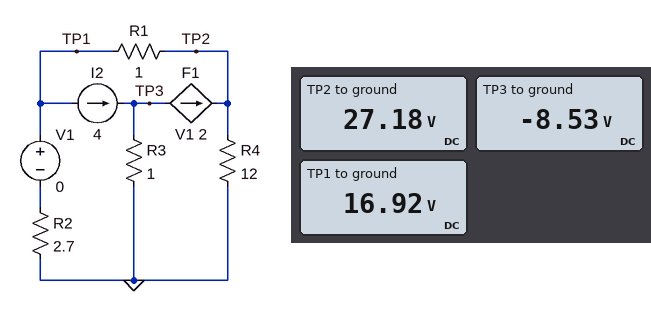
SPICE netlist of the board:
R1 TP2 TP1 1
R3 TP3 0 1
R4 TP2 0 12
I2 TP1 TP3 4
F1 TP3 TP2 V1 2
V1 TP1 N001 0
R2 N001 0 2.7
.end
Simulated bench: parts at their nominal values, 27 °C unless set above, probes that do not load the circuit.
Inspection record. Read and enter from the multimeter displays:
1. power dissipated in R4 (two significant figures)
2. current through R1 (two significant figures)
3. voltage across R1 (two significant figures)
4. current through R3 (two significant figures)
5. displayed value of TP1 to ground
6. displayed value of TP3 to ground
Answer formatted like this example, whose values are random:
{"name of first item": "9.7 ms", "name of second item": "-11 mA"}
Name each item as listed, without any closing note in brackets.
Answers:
{"power dissipated in R4": "62 W", "current through R1": "10 A", "voltage across R1": "10 V", "current through R3": "8.5 A", "displayed value of TP1 to ground": "16.92 V", "displayed value of TP3 to ground": "-8.53 V"}
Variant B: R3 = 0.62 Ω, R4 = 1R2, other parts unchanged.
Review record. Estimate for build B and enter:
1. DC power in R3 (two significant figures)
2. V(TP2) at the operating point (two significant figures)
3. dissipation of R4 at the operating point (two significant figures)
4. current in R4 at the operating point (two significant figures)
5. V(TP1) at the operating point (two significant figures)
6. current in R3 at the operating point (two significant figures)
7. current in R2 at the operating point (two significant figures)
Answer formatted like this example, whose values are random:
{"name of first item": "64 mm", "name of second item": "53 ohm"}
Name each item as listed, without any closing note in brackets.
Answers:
{"DC power in R3": "76 W", "V(TP2) at the operating point": "-9.0 V", "dissipation of R4 at the operating point": "68 W", "current in R4 at the operating point": "7.5 A", "V(TP1) at the operating point": "-9.5 V", "current in R3 at the operating point": "11 A", "current in R2 at the operating point": "3.5 A"}
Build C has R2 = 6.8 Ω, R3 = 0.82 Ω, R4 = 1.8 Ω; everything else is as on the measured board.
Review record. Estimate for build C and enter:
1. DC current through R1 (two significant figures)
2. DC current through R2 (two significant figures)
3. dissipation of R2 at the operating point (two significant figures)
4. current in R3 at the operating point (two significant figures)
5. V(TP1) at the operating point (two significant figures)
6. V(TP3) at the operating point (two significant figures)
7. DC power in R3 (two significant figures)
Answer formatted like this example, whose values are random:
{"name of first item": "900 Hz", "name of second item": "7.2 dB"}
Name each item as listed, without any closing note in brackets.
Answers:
{"DC current through R1": "2.1 A", "DC current through R2": "1.9 A", "dissipation of R2 at the operating point": "24 W", "current in R3 at the operating point": "7.7 A", "V(TP1) at the operating point": "-13 V", "V(TP3) at the operating point": "6.3 V", "DC power in R3": "49 W"}
